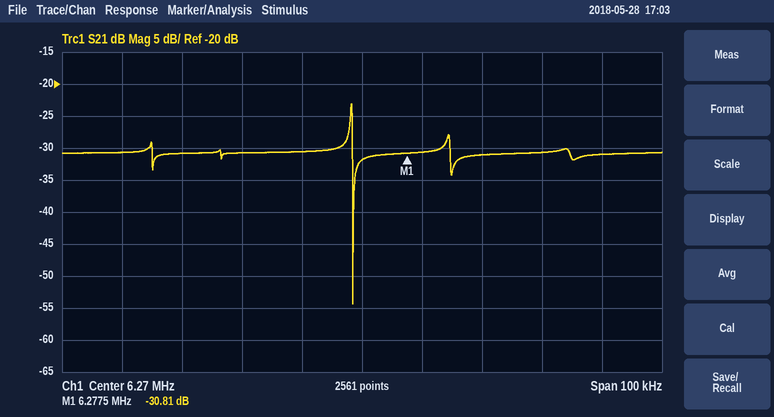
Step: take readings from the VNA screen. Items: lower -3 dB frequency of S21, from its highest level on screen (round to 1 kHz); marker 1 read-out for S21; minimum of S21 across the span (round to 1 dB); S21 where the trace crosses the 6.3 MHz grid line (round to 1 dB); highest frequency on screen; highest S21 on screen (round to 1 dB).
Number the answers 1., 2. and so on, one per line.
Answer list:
1. 6.268 MHz
2. -30.81 dB
3. -54 dB
4. -31 dB
5. 6.32 MHz
6. -23 dB
